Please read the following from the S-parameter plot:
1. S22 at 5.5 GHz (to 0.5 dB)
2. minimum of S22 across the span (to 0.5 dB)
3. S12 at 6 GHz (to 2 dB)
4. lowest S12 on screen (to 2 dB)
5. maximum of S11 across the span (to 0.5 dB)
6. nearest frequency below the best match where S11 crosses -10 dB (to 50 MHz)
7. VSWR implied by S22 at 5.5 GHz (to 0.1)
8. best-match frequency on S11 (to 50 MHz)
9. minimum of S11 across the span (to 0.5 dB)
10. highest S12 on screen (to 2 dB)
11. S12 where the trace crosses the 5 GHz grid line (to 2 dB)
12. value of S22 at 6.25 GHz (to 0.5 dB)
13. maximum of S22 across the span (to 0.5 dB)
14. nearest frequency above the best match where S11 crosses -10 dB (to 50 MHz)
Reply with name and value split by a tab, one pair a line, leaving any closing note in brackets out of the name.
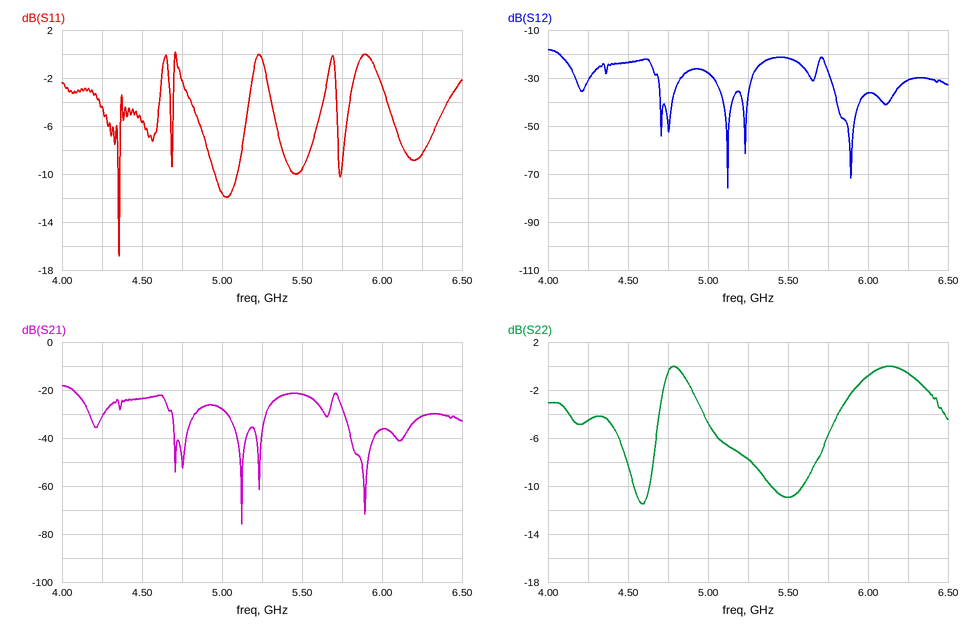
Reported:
S22 at 5.5 GHz	-11.0 dB
minimum of S22 across the span	-11.5 dB
S12 at 6 GHz	-36 dB
lowest S12 on screen	-76 dB
maximum of S11 across the span	0.0 dB
nearest frequency below the best match where S11 crosses -10 dB	4.35 GHz
VSWR implied by S22 at 5.5 GHz	1.8
best-match frequency on S11	4.35 GHz
minimum of S11 across the span	-17.0 dB
highest S12 on screen	-18 dB
S12 where the trace crosses the 5 GHz grid line	-28 dB
value of S22 at 6.25 GHz	-0.5 dB
maximum of S22 across the span	0.0 dB
nearest frequency above the best match where S11 crosses -10 dB	4.35 GHz
